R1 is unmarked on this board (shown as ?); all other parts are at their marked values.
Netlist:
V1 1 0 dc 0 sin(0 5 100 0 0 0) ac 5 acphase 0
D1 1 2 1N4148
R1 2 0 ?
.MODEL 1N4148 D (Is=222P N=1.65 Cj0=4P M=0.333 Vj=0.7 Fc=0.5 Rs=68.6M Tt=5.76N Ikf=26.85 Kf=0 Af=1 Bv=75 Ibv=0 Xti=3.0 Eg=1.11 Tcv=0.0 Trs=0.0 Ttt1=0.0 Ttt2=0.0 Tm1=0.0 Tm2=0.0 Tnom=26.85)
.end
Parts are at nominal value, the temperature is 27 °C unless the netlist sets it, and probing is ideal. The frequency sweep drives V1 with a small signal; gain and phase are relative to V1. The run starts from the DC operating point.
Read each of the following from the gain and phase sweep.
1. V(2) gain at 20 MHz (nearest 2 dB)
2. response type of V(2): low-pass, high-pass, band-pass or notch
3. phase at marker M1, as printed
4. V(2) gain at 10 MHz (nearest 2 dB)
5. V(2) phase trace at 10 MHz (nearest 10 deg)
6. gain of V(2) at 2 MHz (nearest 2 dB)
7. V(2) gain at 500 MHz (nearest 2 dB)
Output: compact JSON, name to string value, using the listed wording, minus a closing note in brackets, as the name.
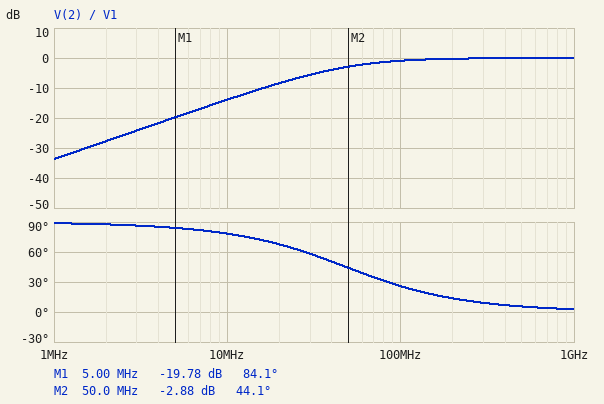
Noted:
{"V(2) gain at 20 MHz": "-8 dB", "response type of V(2): low-pass, high-pass, band-pass or notch": "high-pass", "phase at marker M1, as printed": "84.1 deg", "V(2) gain at 10 MHz": "-14 dB", "V(2) phase trace at 10 MHz": "80 deg", "gain of V(2) at 2 MHz": "-28 dB", "V(2) gain at 500 MHz": "0 dB"}
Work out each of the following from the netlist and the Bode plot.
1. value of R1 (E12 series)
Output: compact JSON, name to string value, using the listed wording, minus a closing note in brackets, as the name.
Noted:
{"value of R1": "820 Ω"}
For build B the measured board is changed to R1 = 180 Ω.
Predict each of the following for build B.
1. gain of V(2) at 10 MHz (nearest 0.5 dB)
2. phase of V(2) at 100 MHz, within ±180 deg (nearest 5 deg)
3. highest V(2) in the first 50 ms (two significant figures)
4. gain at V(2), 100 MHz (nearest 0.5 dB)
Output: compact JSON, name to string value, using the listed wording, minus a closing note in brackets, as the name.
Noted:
{"gain of V(2) at 10 MHz": "-27.0 dB", "phase of V(2) at 100 MHz, within ±180 deg": "65 deg", "highest V(2) in the first 50 ms": "4.2 V", "gain at V(2), 100 MHz": "-7.5 dB"}
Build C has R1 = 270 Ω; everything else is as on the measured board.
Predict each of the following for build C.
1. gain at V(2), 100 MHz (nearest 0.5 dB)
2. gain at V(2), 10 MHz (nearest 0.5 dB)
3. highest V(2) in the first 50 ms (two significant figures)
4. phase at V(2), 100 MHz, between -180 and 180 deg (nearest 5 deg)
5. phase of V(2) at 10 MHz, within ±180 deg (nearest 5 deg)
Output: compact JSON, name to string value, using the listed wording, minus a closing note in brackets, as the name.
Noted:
{"gain at V(2), 100 MHz": "-5.0 dB", "gain at V(2), 10 MHz": "-23.5 dB", "highest V(2) in the first 50 ms": "4.2 V", "phase at V(2), 100 MHz, between -180 and 180 deg": "55 deg", "phase of V(2) at 10 MHz, within ±180 deg": "85 deg"}
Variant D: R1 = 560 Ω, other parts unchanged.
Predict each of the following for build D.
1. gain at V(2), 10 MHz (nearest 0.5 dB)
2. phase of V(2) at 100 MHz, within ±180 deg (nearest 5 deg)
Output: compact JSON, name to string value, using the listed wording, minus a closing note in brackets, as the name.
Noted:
{"gain at V(2), 10 MHz": "-17.0 dB", "phase of V(2) at 100 MHz, within ±180 deg": "35 deg"}
